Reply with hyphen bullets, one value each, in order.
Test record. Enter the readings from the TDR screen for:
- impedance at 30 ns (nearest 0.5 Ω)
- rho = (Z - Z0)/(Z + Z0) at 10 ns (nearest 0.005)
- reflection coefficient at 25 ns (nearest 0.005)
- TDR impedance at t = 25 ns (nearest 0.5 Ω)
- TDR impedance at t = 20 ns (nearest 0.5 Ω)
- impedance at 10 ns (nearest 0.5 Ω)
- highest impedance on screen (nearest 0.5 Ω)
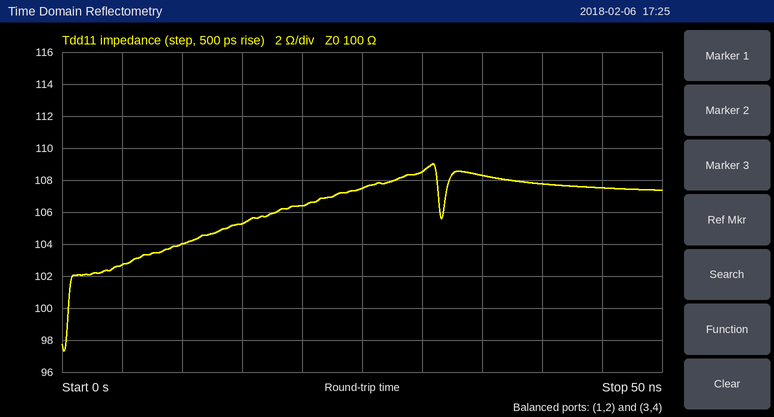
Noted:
- 108.5 Ω
- +0.020
- +0.035
- 107.5 Ω
- 106.5 Ω
- 104.0 Ω
- 109.0 Ω
